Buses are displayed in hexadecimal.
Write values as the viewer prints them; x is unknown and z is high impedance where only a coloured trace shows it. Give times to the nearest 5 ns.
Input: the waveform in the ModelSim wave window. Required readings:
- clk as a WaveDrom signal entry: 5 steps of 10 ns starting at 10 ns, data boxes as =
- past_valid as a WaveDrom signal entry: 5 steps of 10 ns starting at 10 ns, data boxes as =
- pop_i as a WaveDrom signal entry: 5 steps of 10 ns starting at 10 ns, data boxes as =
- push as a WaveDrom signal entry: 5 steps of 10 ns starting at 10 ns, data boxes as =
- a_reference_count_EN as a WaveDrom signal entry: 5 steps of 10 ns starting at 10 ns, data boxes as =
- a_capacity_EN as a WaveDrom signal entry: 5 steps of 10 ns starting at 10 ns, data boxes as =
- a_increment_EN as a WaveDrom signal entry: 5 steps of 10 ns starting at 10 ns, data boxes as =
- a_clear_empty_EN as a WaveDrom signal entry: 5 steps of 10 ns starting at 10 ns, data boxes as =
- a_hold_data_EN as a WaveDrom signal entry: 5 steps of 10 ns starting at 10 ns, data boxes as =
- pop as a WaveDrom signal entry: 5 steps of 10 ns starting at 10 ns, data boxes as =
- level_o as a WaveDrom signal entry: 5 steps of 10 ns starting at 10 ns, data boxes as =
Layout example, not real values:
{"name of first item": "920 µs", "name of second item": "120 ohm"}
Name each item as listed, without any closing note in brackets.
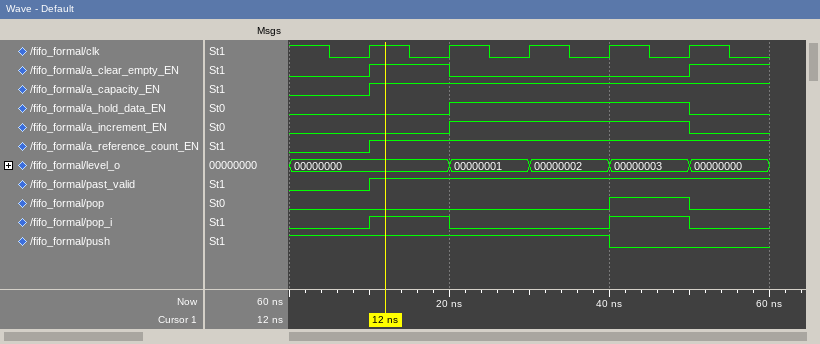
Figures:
{"clk as a WaveDrom signal entry: 5 steps of 10 ns starting at 10 ns, data boxes as =": "{name: 'clk', wave: 'p....'}", "past_valid as a WaveDrom signal entry: 5 steps of 10 ns starting at 10 ns, data boxes as =": "{name: 'past_valid', wave: '1....'}", "pop_i as a WaveDrom signal entry: 5 steps of 10 ns starting at 10 ns, data boxes as =": "{name: 'pop_i', wave: '10.10'}", "push as a WaveDrom signal entry: 5 steps of 10 ns starting at 10 ns, data boxes as =": "{name: 'push', wave: '1..0.'}", "a_reference_count_EN as a WaveDrom signal entry: 5 steps of 10 ns starting at 10 ns, data boxes as =": "{name: 'a_reference_count_EN', wave: '1....'}", "a_capacity_EN as a WaveDrom signal entry: 5 steps of 10 ns starting at 10 ns, data boxes as =": "{name: 'a_capacity_EN', wave: '1....'}", "a_increment_EN as a WaveDrom signal entry: 5 steps of 10 ns starting at 10 ns, data boxes as =": "{name: 'a_increment_EN', wave: '01..0'}", "a_clear_empty_EN as a WaveDrom signal entry: 5 steps of 10 ns starting at 10 ns, data boxes as =": "{name: 'a_clear_empty_EN', wave: '10..1'}", "a_hold_data_EN as a WaveDrom signal entry: 5 steps of 10 ns starting at 10 ns, data boxes as =": "{name: 'a_hold_data_EN', wave: '01..0'}", "pop as a WaveDrom signal entry: 5 steps of 10 ns starting at 10 ns, data boxes as =": "{name: 'pop', wave: '0..10'}", "level_o as a WaveDrom signal entry: 5 steps of 10 ns starting at 10 ns, data boxes as =": "{name: 'level_o', wave: '=====', data: '00000000 00000001 00000002 00000003 00000000'}"}
